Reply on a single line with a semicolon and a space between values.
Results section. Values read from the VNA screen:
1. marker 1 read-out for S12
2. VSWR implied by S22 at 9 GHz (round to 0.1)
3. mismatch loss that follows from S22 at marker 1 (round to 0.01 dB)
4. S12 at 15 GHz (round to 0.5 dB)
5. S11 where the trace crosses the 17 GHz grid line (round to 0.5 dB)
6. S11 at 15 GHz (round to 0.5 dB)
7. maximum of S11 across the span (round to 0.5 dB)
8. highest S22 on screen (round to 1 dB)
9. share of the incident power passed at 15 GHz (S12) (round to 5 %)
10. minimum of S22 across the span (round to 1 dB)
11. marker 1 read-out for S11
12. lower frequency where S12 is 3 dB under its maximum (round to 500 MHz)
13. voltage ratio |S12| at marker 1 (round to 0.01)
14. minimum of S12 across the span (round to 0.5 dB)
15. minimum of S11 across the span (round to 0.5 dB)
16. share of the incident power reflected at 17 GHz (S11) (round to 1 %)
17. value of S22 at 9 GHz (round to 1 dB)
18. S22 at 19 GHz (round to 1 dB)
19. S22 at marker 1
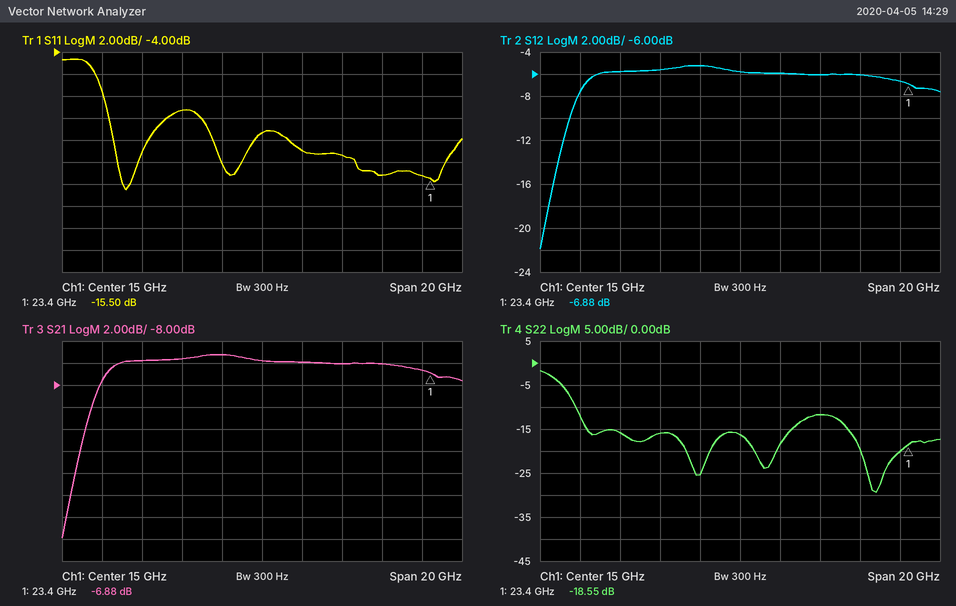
-6.88 dB; 1.4; 0.06 dB; -6.0 dB; -13.0 dB; -11.5 dB; -4.5 dB; -2 dB; 25 %; -29 dB; -15.50 dB; 7.0 GHz; 0.45; -22.0 dB; -16.5 dB; 5 %; -16 dB; -12 dB; -18.55 dB
